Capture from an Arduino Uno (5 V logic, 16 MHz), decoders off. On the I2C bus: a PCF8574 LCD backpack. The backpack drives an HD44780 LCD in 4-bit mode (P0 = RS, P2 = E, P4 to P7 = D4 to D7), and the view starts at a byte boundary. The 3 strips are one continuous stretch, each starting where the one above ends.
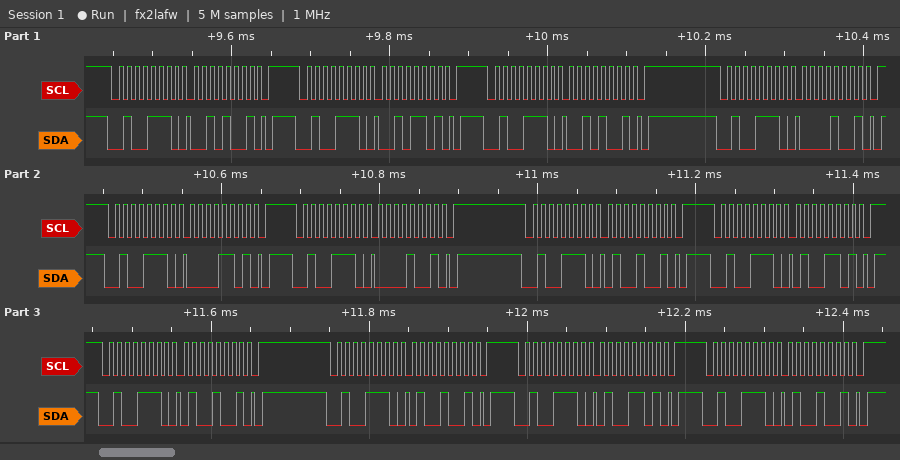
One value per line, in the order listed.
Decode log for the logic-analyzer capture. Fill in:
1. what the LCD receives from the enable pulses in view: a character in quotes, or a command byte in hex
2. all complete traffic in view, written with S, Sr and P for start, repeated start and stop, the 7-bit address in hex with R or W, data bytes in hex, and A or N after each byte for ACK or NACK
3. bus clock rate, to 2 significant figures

' ' 'D'
S 27W A 29 A P S 27W A 2D A P S 27W A 29 A P S 27W A 09 A P S 27W A 0D A P S 27W A 09 A P S 27W A 49 A P S 27W A 4D A P S 27W A 49 A P S 27W A 49 A P S 27W A 4D A P S 27W A 49 A P
100 kHz
